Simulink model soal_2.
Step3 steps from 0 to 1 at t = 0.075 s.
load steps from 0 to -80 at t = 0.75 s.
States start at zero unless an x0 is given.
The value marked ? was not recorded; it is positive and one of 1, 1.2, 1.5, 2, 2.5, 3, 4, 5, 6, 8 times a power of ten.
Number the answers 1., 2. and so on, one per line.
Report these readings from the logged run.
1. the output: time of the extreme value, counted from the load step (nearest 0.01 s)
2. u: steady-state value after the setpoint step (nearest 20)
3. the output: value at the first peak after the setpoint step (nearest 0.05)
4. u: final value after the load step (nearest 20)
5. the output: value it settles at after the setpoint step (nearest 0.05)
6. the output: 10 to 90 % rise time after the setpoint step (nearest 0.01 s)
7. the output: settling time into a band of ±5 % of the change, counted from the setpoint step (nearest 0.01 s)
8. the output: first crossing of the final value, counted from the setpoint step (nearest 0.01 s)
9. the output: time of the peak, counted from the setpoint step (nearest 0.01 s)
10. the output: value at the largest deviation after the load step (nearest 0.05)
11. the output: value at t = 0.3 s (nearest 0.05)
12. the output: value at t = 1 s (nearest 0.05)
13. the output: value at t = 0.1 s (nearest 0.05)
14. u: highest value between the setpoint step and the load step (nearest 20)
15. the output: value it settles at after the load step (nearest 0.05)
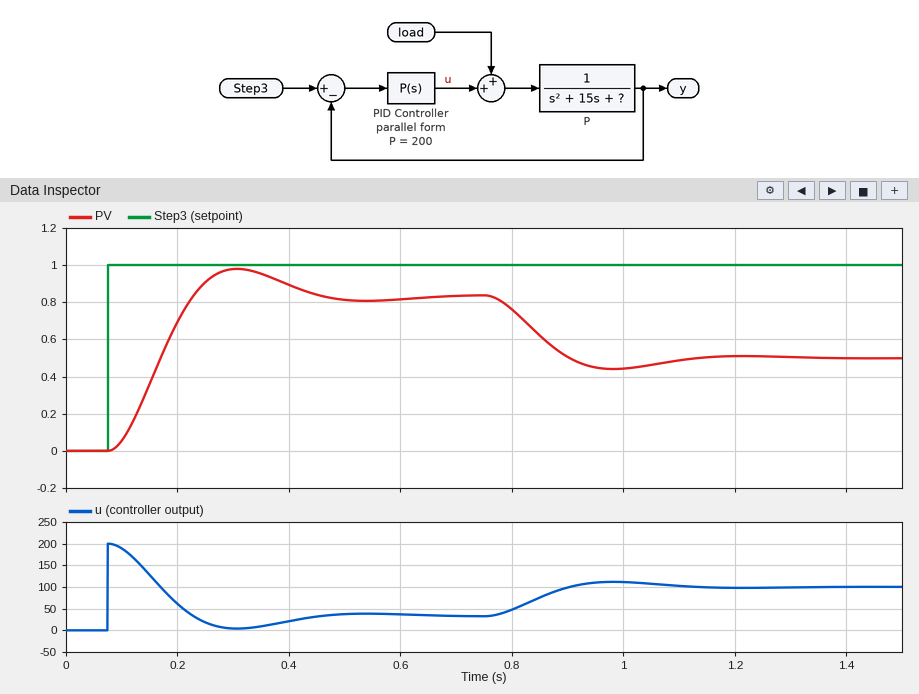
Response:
1. 0.23 s
2. 40
3. 1.00
4. 100
5. 0.85
6. 0.10 s
7. 0.34 s
8. 0.15 s
9. 0.23 s
10. 0.45
11. 1.00
12. 0.45
13. 0.05
14. 200
15. 0.50
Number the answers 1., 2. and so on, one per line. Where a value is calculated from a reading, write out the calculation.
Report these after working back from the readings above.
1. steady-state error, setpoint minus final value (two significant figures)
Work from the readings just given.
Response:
1. 1 - 0.85 = 0.15
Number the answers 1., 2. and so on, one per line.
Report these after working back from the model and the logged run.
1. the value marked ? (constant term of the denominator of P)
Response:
1. 40
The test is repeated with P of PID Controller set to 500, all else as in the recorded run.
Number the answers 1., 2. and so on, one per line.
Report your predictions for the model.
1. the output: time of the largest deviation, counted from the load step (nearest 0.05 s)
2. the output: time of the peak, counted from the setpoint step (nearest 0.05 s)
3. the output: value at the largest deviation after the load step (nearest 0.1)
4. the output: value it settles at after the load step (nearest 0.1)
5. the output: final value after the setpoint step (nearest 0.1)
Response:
1. 0.15 s
2. 0.15 s
3. 0.7
4. 0.8
5. 0.9
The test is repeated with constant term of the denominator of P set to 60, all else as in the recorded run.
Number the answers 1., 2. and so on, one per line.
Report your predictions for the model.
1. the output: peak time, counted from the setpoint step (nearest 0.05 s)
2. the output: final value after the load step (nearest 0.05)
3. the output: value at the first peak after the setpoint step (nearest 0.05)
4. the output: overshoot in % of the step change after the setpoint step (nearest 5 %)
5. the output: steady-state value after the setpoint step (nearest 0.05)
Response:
1. 0.20 s
2. 0.45
3. 0.90
4. 20 %
5. 0.75
